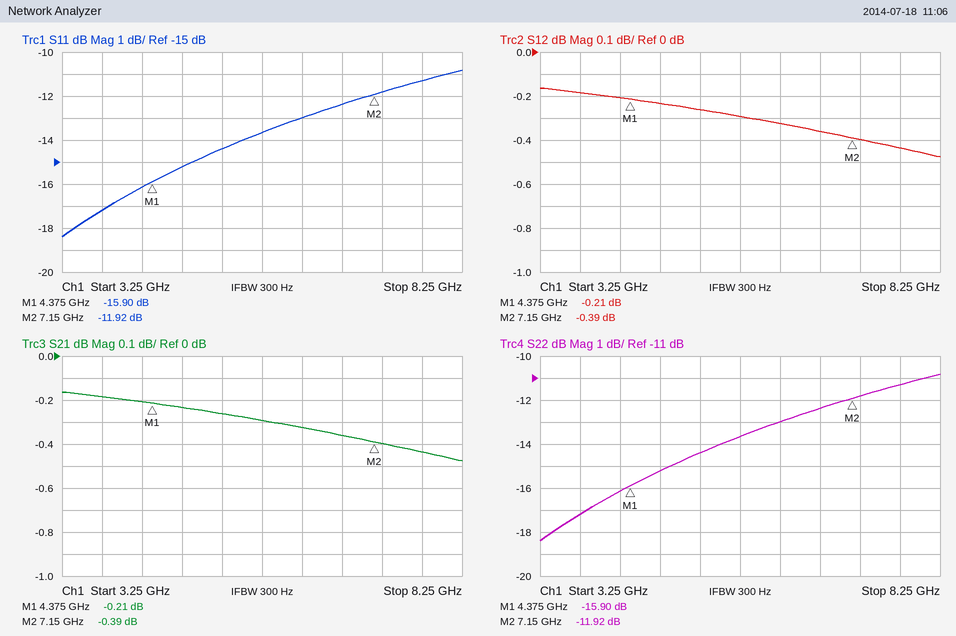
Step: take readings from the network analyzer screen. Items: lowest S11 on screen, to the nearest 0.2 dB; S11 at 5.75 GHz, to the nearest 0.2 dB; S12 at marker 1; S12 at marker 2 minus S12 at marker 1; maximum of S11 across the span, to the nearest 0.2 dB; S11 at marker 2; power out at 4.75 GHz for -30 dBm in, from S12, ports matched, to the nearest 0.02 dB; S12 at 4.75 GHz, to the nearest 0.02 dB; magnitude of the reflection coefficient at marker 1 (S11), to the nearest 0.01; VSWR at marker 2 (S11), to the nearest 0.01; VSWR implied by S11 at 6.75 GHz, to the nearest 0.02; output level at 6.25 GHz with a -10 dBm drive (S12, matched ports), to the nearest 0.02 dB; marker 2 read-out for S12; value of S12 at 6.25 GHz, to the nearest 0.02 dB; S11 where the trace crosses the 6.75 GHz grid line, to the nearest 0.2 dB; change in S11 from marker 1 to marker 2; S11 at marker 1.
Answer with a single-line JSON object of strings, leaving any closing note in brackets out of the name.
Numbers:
{"lowest S11 on screen, to the nearest 0.2 dB": "-18.4 dB", "S11 at 5.75 GHz, to the nearest 0.2 dB": "-13.6 dB", "S12 at marker 1": "-0.21 dB", "S12 at marker 2 minus S12 at marker 1": "-0.18 dB", "maximum of S11 across the span, to the nearest 0.2 dB": "-10.8 dB", "S11 at marker 2": "-11.92 dB", "power out at 4.75 GHz for -30 dBm in, from S12, ports matched, to the nearest 0.02 dB": "-30.24 dBm", "S12 at 4.75 GHz, to the nearest 0.02 dB": "-0.24 dB", "magnitude of the reflection coefficient at marker 1 (S11), to the nearest 0.01": "0.16", "VSWR at marker 2 (S11), to the nearest 0.01": "1.68", "VSWR implied by S11 at 6.75 GHz, to the nearest 0.02": "1.64", "output level at 6.25 GHz with a -10 dBm drive (S12, matched ports), to the nearest 0.02 dB": "-10.32 dBm", "marker 2 read-out for S12": "-0.39 dB", "value of S12 at 6.25 GHz, to the nearest 0.02 dB": "-0.32 dB", "S11 where the trace crosses the 6.75 GHz grid line, to the nearest 0.2 dB": "-12.4 dB", "change in S11 from marker 1 to marker 2": "3.98 dB", "S11 at marker 1": "-15.90 dB"}
